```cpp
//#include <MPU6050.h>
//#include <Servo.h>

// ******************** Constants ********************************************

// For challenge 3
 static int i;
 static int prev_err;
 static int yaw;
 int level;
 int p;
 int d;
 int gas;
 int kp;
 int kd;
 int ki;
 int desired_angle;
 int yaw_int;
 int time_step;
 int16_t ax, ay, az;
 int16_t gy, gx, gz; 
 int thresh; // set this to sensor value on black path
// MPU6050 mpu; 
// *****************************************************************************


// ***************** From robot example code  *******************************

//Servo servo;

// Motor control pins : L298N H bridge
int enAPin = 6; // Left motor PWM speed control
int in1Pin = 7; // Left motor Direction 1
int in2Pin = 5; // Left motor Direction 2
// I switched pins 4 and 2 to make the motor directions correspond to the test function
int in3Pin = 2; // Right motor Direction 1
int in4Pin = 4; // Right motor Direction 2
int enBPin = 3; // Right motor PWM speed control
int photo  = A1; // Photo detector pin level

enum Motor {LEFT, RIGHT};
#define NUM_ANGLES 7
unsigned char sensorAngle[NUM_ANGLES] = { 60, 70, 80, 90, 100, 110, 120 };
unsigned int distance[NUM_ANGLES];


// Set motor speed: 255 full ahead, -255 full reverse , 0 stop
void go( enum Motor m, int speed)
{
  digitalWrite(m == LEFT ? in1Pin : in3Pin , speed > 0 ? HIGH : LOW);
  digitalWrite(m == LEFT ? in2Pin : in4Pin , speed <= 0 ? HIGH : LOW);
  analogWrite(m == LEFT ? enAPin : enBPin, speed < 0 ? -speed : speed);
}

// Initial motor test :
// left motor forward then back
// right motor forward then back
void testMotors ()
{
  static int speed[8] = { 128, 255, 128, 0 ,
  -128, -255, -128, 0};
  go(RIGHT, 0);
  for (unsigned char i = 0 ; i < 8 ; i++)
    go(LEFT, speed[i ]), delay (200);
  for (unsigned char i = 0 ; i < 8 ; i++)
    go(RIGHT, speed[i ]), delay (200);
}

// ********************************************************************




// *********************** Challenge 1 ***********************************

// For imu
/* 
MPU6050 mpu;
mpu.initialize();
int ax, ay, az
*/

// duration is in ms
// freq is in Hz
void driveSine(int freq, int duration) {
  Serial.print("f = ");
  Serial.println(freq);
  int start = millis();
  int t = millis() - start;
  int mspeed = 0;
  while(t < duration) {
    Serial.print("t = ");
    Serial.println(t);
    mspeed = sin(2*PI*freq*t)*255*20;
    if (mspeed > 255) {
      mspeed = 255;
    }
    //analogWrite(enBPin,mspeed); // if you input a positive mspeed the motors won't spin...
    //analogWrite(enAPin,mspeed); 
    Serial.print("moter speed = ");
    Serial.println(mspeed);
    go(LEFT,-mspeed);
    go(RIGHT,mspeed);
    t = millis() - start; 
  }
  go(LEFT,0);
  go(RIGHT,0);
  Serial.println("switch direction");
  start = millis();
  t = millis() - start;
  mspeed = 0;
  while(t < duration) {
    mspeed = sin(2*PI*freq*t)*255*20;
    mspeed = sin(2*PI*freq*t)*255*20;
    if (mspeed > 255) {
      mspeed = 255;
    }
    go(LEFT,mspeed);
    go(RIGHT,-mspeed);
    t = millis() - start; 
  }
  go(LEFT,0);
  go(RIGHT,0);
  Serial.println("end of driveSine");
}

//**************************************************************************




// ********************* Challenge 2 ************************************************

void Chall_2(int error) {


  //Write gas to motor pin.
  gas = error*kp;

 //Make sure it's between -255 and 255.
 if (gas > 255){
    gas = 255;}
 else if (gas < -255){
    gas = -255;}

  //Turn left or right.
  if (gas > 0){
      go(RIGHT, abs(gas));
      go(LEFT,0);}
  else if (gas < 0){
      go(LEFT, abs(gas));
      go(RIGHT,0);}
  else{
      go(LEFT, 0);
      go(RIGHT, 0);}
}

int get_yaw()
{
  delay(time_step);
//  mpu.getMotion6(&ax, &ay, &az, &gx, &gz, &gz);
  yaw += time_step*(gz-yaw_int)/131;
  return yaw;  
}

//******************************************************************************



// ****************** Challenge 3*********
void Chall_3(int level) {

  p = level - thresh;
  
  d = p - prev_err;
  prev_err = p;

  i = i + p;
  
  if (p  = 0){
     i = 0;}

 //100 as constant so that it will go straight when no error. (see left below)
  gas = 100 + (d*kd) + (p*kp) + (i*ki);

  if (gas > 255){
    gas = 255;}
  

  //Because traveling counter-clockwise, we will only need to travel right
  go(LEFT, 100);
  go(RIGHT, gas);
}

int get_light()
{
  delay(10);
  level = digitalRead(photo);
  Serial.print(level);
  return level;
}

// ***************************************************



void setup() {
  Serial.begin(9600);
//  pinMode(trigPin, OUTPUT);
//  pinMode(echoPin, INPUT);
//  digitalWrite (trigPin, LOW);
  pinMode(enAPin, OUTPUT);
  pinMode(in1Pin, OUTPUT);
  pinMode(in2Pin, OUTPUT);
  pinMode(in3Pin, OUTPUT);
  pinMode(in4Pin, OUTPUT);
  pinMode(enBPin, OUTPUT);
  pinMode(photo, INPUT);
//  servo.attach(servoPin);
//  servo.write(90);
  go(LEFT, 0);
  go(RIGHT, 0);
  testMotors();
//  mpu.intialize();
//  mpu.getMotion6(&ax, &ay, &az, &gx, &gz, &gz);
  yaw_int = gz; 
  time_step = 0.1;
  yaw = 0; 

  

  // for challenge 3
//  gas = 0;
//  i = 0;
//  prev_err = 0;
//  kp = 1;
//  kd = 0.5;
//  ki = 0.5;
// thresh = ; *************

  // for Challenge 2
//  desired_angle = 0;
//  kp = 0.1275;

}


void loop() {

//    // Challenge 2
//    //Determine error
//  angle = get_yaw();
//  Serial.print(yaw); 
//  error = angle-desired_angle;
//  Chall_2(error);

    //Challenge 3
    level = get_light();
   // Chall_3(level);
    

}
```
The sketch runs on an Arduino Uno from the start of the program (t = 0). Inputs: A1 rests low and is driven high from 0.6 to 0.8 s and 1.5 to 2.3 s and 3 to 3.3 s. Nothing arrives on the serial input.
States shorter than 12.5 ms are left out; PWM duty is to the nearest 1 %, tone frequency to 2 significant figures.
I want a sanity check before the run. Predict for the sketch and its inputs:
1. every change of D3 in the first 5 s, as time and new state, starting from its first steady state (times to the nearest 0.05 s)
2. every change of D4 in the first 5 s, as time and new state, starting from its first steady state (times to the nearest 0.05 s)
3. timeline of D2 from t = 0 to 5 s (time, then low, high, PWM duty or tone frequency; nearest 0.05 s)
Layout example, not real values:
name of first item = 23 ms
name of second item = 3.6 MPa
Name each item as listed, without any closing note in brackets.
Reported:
every change of D3 in the first 5 s, as time and new state, starting from its first steady state = 0 s low; 1.6 s PWM 50 %; 1.8 s high; 2 s PWM 50 %; 2.2 s low; 2.4 s PWM 50 %; 2.6 s high; 2.8 s PWM 50 %; 3 s low
every change of D4 in the first 5 s, as time and new state, starting from its first steady state = 0 s high; 1.6 s low; 2.2 s high
timeline of D2 from t = 0 to 5 s = 0 s low; 1.6 s high; 2.2 s low
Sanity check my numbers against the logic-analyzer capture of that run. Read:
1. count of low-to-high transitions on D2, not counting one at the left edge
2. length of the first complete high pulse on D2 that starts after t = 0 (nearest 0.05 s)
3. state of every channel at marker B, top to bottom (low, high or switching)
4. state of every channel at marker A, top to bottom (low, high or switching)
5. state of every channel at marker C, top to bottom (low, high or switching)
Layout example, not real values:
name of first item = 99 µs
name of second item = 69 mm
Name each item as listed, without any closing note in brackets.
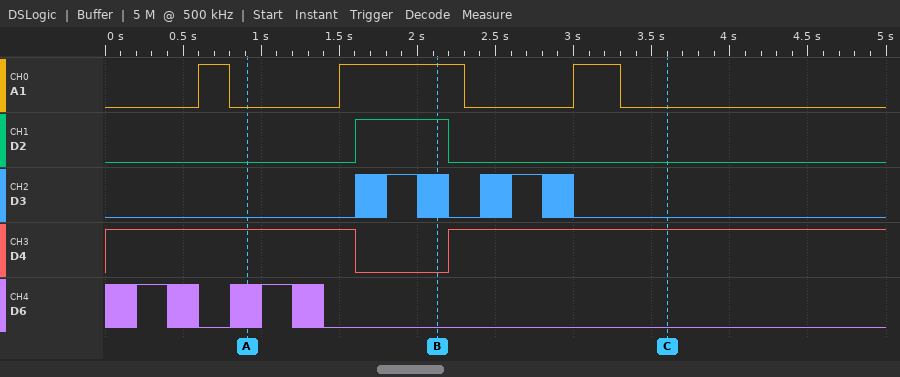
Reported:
count of low-to-high transitions on D2, not counting one at the left edge = 1
length of the first complete high pulse on D2 that starts after t = 0 = 0.60 s
state of every channel at marker B, top to bottom = A1 high, D2 high, D3 switching, D4 low, D6 low
state of every channel at marker A, top to bottom = A1 low, D2 low, D3 low, D4 high, D6 switching
state of every channel at marker C, top to bottom = A1 low, D2 low, D3 low, D4 high, D6 low
